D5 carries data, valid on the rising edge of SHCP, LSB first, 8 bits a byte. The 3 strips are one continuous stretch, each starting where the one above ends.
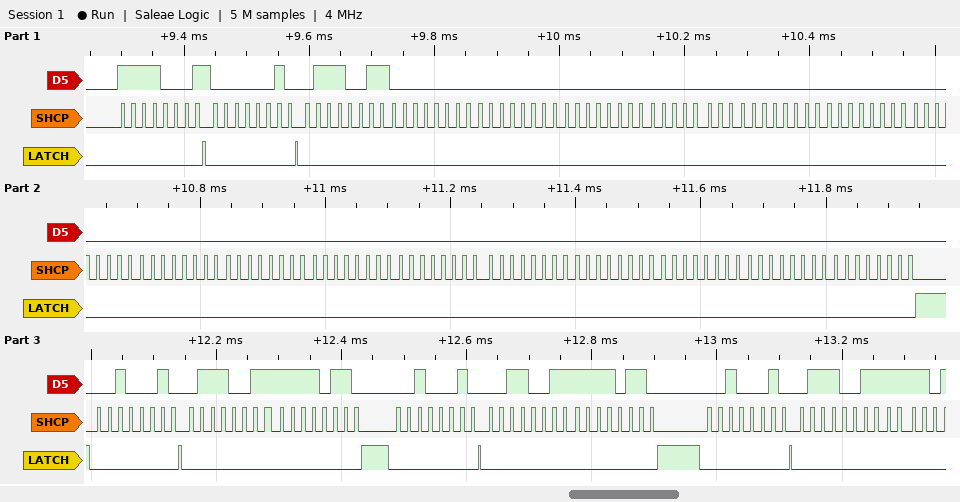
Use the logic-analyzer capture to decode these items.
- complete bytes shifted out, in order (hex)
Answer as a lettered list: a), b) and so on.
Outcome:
a) 8F 40 CE 00 00 00 00 00 00 00 00 00 00 00 00 00 00 00 00 44 CE 6F 44 CC 6F 44 CE
